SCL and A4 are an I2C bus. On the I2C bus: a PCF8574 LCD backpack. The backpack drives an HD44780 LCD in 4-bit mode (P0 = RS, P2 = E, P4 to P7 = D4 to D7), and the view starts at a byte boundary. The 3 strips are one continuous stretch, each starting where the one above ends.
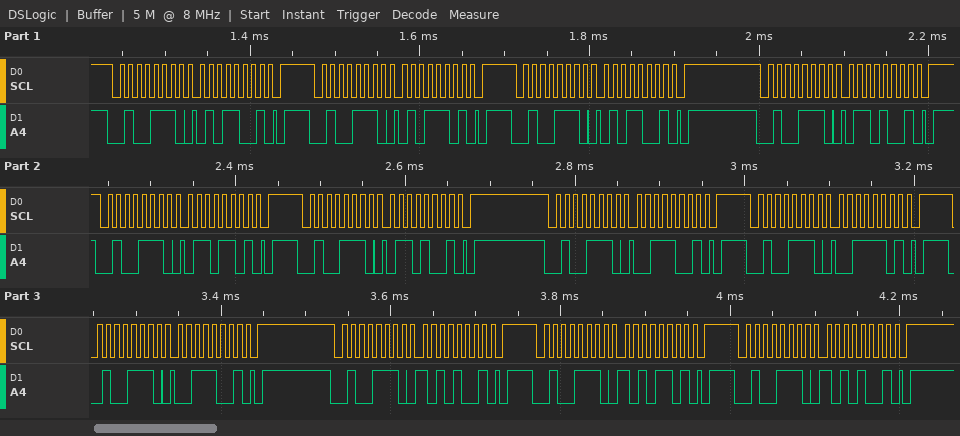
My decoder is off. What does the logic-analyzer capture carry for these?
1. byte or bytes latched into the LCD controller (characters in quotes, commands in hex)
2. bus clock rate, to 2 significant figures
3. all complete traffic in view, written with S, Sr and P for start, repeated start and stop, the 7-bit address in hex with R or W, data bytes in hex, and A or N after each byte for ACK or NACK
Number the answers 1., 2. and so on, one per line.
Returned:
1. 'V' ':'
2. 100 kHz
3. S 27W A 59 A P S 27W A 5D A P S 27W A 59 A P S 27W A 69 A P S 27W A 6D A P S 27W A 69 A P S 27W A 39 A P S 27W A 3D A P S 27W A 39 A P S 27W A A9 A P S 27W A AD A P S 27W A A9 A P
